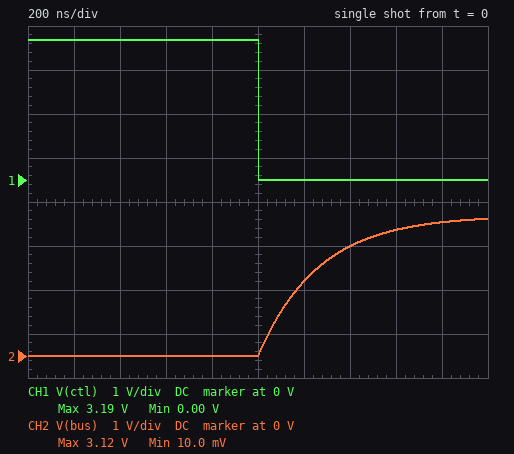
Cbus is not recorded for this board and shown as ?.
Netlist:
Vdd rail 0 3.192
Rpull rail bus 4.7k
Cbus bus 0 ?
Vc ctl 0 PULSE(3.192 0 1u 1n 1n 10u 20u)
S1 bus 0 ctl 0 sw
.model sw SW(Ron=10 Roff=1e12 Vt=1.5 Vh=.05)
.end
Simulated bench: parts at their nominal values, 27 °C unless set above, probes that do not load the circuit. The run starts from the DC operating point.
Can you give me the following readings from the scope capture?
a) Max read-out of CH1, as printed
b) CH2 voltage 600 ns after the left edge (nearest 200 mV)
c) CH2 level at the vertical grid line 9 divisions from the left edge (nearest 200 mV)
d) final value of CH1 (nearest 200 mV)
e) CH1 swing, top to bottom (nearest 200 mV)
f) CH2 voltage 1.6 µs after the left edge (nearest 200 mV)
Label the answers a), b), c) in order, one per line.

a) 3.19 V
b) 0 V
c) 3.0 V
d) 0 V
e) 3.2 V
f) 2.8 V
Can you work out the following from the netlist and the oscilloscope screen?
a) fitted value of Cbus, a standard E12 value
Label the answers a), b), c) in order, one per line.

a) 56 pF
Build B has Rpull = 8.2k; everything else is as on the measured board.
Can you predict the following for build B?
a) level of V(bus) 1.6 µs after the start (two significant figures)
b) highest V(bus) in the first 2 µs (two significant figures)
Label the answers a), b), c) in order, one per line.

a) 2.3 V
b) 2.8 V
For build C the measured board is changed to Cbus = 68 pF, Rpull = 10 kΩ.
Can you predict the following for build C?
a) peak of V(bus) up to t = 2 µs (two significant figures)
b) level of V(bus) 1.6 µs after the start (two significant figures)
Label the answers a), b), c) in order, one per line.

a) 2.5 V
b) 1.9 V
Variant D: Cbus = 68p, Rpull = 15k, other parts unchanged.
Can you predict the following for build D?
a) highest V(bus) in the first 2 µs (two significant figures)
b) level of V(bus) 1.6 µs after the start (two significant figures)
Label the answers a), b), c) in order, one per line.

a) 2.0 V
b) 1.4 V
